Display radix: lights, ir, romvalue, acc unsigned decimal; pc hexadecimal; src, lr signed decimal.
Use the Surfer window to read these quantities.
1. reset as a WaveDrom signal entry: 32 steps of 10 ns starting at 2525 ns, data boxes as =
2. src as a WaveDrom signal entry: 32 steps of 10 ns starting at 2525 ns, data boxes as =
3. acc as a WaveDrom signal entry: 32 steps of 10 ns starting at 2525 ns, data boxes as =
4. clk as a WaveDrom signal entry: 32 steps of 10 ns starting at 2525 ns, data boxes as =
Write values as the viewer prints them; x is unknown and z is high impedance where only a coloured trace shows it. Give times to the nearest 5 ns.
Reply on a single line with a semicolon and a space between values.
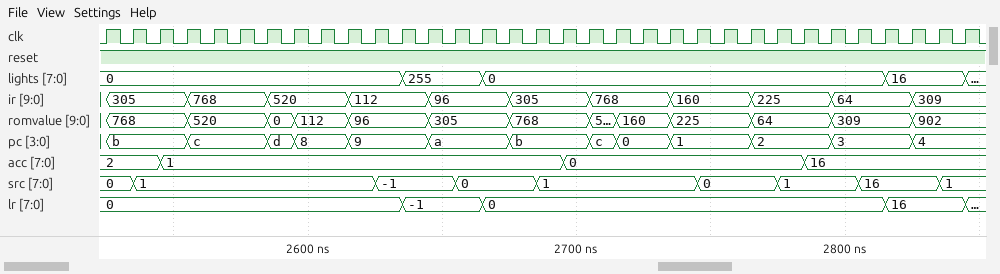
{name: 'reset', wave: '1...............................'}; {name: 'src', wave: '==........=..=..=.....=..=..=..=', data: '0 1 -1 0 1 0 1 16 1'}; {name: 'acc', wave: '=.=..............=........=.....', data: '2 1 0 16'}; {name: 'clk', wave: 'p...............................'}
